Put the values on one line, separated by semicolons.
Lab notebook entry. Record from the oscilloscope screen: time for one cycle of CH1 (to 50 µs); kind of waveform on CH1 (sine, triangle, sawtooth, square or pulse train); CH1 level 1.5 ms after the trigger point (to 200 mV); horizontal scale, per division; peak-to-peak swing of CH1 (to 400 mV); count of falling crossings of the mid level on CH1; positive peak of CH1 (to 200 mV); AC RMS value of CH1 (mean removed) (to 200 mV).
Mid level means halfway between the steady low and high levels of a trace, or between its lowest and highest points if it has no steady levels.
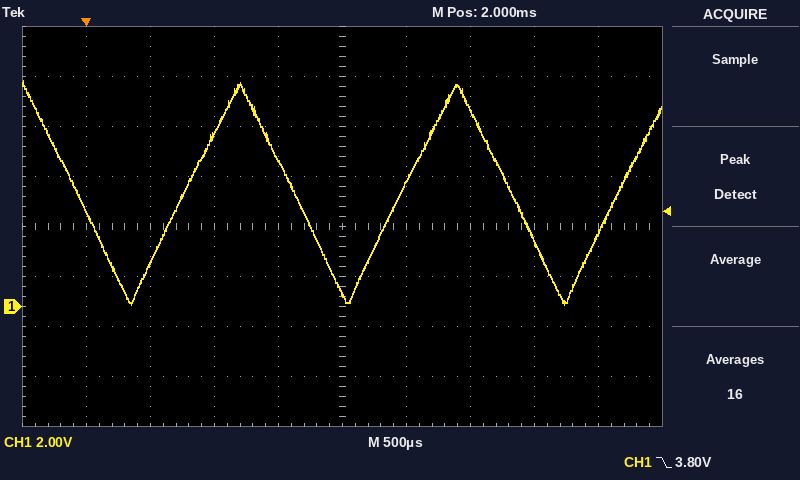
1.70 ms; triangle; 5.8 V; 500 µs; 8.8 V; 3; 9.0 V; 2.6 V
